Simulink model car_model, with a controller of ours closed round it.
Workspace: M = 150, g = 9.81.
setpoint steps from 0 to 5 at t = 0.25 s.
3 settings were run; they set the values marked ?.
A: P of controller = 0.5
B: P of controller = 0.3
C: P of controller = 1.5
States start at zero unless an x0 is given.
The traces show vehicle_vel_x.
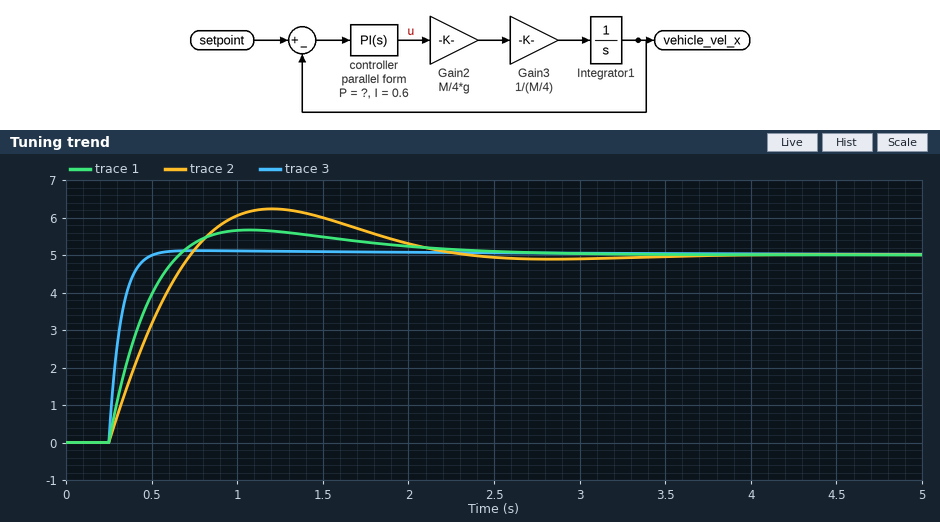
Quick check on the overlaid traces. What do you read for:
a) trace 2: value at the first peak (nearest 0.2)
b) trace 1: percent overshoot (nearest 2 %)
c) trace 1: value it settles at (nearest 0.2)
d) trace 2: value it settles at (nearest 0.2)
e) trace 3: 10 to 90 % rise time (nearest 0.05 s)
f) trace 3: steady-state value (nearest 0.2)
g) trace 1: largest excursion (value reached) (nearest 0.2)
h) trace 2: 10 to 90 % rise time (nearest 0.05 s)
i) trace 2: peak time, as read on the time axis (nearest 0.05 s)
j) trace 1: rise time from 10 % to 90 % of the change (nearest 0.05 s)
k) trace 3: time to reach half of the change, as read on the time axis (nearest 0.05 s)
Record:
6.2
14 %
5.0
5.0
0.15 s
5.0
5.6
0.35 s
1.20 s
0.30 s
0.30 s
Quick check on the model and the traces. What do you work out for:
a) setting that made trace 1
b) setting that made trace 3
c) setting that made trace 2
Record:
A
C
B
